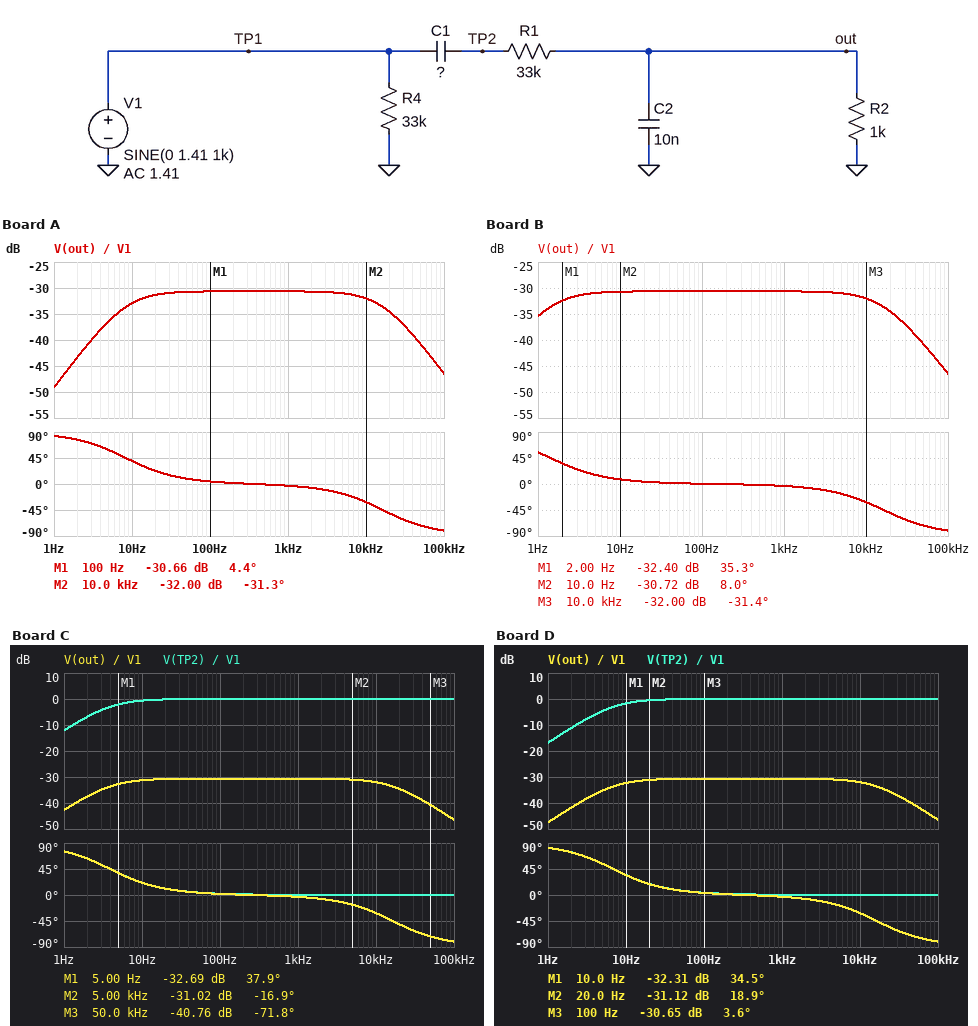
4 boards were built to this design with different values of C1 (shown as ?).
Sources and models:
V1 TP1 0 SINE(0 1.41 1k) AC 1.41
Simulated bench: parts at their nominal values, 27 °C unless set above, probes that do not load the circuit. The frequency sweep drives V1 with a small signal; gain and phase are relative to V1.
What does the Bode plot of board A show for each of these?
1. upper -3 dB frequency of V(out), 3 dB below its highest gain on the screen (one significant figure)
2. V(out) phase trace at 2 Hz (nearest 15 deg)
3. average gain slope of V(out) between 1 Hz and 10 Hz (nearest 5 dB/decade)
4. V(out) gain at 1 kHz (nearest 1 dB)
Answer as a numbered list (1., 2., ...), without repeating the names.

1. 20 kHz
2. 75 deg
3. 15 dB/decade
4. -31 dB
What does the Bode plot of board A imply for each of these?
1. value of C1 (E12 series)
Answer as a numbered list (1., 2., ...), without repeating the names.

1. 560 nF
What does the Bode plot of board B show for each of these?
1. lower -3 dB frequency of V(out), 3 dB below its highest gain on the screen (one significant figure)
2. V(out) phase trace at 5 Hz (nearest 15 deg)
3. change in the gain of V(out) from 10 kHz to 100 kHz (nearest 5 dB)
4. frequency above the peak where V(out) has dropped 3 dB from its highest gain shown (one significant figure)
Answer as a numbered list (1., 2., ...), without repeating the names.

1. 1 Hz
2. 15 deg
3. -15 dB
4. 20 kHz
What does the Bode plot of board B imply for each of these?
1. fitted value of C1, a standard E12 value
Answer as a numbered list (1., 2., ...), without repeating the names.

1. 3.3 µF
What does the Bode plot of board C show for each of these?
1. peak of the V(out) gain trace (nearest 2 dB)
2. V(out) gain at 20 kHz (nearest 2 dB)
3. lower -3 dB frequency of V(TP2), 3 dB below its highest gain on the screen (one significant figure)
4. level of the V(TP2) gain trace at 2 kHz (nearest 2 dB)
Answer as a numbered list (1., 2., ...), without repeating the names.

1. -30 dB
2. -34 dB
3. 4 Hz
4. 0 dB
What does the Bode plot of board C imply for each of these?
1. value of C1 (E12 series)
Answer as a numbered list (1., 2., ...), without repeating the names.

1. 1.2 µF
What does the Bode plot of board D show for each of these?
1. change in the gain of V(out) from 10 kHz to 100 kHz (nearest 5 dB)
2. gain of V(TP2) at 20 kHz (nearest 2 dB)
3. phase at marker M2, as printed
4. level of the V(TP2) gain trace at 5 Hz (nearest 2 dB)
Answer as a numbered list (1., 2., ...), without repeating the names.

1. -15 dB
2. 0 dB
3. 18.9 deg
4. -4 dB
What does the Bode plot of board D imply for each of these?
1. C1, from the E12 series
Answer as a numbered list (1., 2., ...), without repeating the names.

1. 680 nF
